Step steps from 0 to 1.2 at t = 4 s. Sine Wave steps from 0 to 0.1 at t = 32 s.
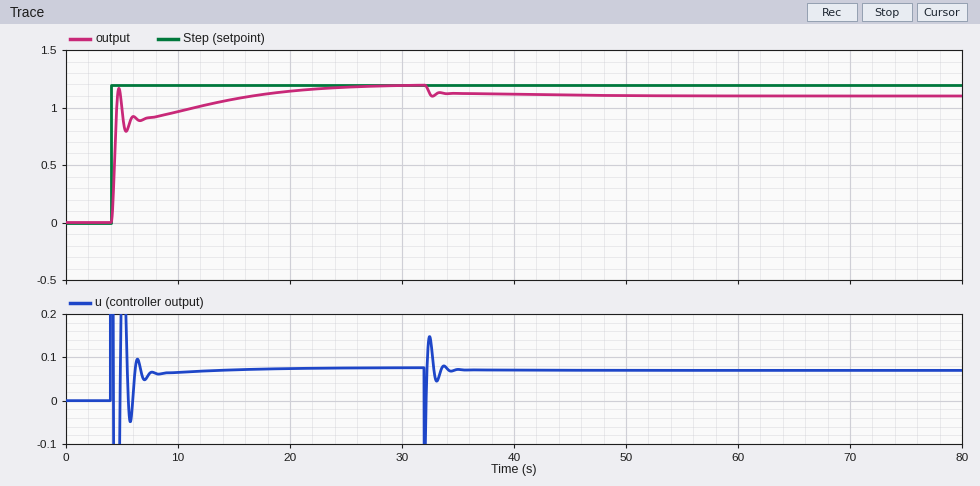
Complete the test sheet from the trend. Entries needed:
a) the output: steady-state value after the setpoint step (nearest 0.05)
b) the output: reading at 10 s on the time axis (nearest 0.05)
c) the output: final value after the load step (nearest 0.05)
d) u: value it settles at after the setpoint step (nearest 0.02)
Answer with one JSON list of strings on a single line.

["1.20", "0.95", "1.10", "0.08"]
